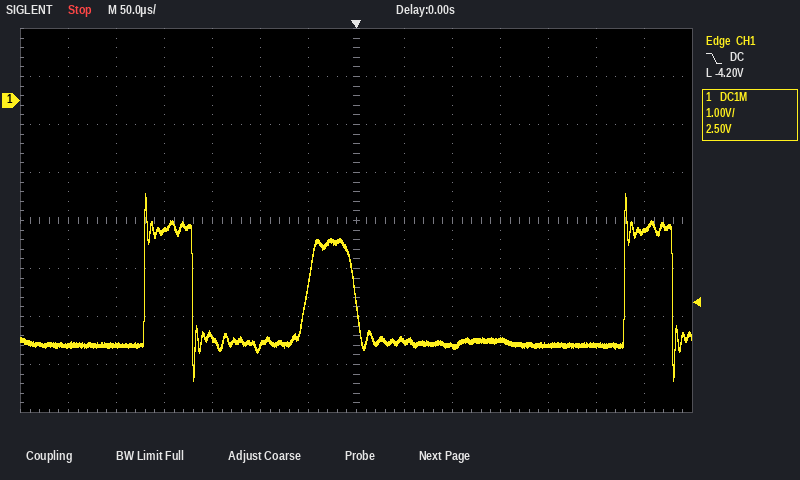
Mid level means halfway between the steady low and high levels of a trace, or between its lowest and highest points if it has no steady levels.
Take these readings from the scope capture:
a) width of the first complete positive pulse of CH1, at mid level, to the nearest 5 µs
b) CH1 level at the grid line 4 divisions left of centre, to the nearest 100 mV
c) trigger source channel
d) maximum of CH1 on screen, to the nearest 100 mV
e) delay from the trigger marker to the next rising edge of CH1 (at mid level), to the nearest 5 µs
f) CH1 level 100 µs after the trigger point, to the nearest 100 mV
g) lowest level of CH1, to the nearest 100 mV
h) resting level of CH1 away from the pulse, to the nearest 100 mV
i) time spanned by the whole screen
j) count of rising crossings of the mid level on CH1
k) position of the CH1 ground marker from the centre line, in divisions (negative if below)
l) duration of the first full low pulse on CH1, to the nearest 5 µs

50 µs
-2.7 V
CH1
-1.9 V
280 µs
-5.1 V
-5.9 V
-5.1 V
700 µs
3
+2.5 div
120 µs
